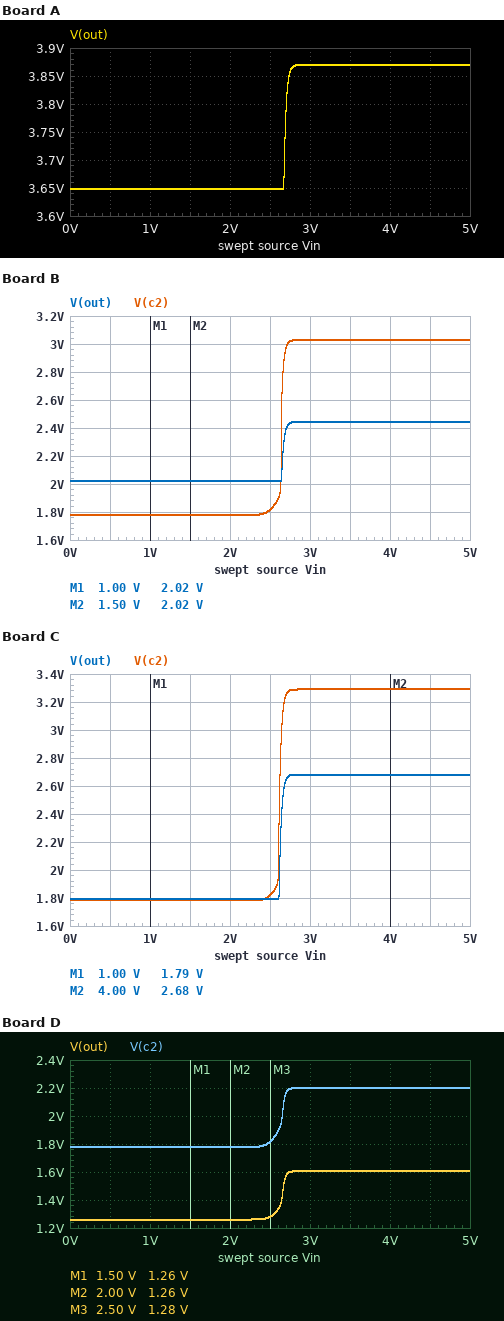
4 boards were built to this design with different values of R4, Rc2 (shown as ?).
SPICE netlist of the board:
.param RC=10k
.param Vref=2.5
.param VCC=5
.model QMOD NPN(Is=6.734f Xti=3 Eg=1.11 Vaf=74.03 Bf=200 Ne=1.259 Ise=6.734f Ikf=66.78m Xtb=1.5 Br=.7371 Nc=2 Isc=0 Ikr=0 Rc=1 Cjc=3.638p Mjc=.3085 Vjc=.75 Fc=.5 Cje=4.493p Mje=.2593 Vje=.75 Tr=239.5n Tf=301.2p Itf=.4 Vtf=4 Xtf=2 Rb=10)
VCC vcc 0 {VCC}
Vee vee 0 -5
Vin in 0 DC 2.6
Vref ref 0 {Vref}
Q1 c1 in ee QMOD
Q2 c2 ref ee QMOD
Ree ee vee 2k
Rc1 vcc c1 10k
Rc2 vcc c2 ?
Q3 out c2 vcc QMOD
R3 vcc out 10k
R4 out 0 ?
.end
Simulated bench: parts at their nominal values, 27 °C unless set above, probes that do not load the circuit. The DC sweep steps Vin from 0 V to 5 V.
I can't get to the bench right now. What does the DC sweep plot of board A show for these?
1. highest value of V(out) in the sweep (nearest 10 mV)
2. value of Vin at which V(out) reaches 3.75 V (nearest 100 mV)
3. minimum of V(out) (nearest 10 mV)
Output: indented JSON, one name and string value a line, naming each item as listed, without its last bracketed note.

{
  "highest value of V(out) in the sweep": "3.87 V",
  "value of Vin at which V(out) reaches 3.75 V": "2.7 V",
  "minimum of V(out)": "3.65 V"
}
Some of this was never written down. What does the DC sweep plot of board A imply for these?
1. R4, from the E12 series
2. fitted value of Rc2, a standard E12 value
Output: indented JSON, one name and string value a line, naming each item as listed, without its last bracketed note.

{
  "R4, from the E12 series": "27 kΩ",
  "fitted value of Rc2, a standard E12 value": "33 kΩ"
}
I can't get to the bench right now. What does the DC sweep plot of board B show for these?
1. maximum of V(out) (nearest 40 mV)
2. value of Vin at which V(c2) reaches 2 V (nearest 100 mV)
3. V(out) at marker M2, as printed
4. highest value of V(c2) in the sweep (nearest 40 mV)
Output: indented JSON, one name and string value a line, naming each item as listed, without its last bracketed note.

{
  "maximum of V(out)": "2.44 V",
  "value of Vin at which V(c2) reaches 2 V": "2.6 V",
  "V(out) at marker M2, as printed": "2.02 V",
  "highest value of V(c2) in the sweep": "3.04 V"
}
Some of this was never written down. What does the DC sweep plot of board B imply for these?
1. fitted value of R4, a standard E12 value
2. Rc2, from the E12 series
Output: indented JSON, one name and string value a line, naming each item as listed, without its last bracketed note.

{
  "fitted value of R4, a standard E12 value": "6.8 kΩ",
  "Rc2, from the E12 series": "33 kΩ"
}
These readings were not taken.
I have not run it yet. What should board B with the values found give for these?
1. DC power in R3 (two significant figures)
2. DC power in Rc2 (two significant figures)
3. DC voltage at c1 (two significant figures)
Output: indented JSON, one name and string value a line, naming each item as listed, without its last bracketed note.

{
  "DC power in R3": "890 µW",
  "DC power in Rc2": "290 µW",
  "DC voltage at c1": "1.9 V"
}
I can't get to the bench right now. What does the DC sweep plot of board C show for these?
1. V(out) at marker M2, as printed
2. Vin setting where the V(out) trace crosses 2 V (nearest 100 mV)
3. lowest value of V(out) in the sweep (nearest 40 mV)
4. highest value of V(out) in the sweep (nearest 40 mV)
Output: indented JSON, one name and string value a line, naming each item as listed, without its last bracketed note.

{
  "V(out) at marker M2, as printed": "2.68 V",
  "Vin setting where the V(out) trace crosses 2 V": "2.6 V",
  "lowest value of V(out) in the sweep": "1.80 V",
  "highest value of V(out) in the sweep": "2.68 V"
}
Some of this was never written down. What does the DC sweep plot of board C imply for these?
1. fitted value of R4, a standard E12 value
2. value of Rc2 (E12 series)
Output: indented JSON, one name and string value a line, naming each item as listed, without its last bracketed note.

{
  "fitted value of R4, a standard E12 value": "5.6 kΩ",
  "value of Rc2": "12 kΩ"
}
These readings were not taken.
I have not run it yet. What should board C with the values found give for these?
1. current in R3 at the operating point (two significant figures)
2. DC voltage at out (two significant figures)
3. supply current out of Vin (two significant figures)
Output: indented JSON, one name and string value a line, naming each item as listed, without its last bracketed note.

{
  "current in R3 at the operating point": "320 µA",
  "DC voltage at out": "1.8 V",
  "supply current out of Vin": "2.8 mA"
}
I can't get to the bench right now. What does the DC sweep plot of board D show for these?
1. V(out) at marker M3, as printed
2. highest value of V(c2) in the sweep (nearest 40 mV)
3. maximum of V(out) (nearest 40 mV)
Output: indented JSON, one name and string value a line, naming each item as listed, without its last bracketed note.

{
  "V(out) at marker M3, as printed": "1.28 V",
  "highest value of V(c2) in the sweep": "2.20 V",
  "maximum of V(out)": "1.60 V"
}
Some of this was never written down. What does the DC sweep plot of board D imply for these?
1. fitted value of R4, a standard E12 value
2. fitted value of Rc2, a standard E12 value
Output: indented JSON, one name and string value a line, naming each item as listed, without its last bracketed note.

{
  "fitted value of R4, a standard E12 value": "3.3 kΩ",
  "fitted value of Rc2, a standard E12 value": "33 kΩ"
}
